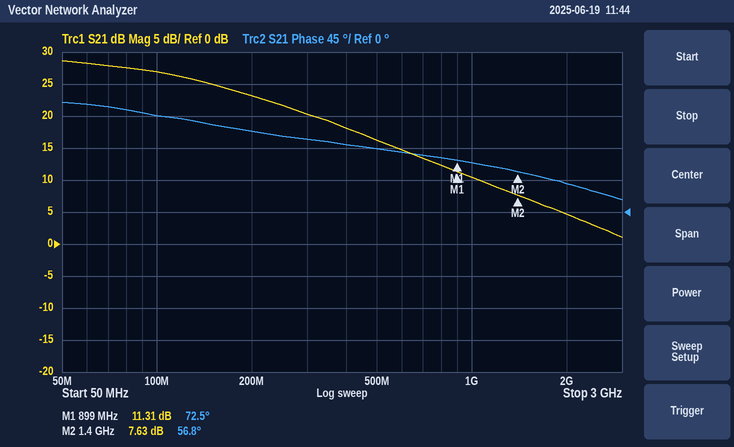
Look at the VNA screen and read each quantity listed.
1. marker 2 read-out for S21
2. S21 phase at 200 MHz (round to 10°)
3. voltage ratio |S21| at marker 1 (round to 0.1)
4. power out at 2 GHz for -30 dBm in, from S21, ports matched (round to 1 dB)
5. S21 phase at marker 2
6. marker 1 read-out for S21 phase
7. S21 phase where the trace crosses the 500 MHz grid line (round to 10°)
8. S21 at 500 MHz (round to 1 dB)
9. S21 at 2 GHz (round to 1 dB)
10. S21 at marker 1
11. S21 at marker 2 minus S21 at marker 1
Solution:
7.63 dB
110°
3.7
-25 dBm
56.8°
72.5°
90°
16 dB
5 dB
11.31 dB
-3.68 dB
